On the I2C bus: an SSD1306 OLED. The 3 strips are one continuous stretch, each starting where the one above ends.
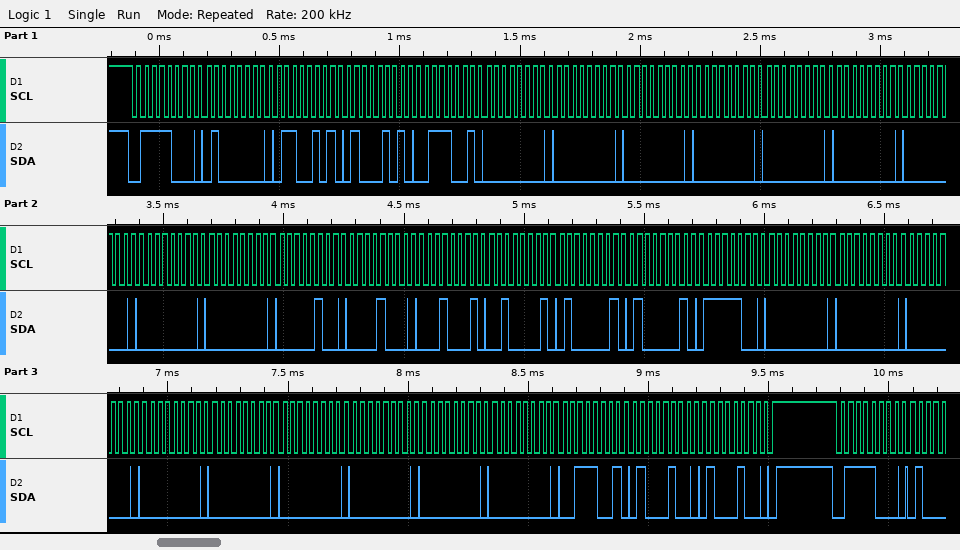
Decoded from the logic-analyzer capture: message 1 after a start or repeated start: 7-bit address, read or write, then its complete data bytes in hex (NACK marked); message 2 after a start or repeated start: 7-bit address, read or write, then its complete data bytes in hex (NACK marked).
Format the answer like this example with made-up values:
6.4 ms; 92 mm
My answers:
0x3C write: 40 65 45 39 00 00 00 00 00 00 00 00 00 04 08 11 21 41 41 7C 00 00 00 00 00 00 00 00 00 39 44 44; 0x3C write
